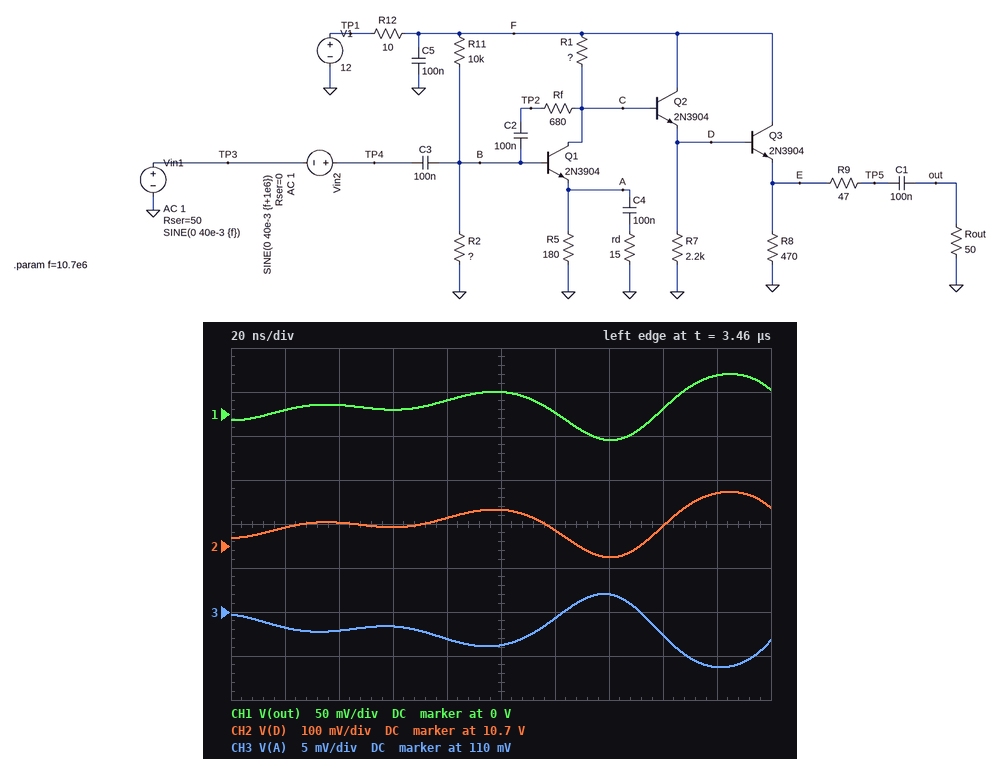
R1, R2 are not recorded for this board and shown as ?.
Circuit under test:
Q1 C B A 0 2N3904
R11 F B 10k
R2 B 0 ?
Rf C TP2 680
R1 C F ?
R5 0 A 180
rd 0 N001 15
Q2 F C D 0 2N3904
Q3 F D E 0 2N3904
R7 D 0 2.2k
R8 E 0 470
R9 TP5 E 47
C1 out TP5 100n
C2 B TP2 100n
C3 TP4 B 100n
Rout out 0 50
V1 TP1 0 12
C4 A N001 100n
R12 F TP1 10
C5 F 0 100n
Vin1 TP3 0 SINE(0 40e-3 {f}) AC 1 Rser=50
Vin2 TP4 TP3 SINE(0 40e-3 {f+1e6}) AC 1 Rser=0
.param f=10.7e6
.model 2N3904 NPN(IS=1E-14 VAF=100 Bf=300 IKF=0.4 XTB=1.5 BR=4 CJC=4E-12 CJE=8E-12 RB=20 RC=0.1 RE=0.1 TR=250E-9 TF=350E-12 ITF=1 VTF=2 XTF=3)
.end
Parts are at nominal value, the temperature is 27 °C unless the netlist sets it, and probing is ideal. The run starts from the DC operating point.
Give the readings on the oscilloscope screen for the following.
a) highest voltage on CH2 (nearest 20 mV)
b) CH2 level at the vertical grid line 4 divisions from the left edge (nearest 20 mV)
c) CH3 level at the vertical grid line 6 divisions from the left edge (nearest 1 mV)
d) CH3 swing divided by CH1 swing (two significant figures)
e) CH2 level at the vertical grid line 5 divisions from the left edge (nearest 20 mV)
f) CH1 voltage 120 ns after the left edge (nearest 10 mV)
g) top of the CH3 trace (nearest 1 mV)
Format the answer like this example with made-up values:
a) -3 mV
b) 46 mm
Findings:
a) 10.82 V
b) 10.76 V
c) 109 mV
d) 0.11
e) 10.78 V
f) 0 V
g) 112 mV
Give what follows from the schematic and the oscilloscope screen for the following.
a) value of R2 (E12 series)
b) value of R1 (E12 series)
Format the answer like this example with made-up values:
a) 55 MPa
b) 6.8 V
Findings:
a) 680 Ω
b) 470 Ω
